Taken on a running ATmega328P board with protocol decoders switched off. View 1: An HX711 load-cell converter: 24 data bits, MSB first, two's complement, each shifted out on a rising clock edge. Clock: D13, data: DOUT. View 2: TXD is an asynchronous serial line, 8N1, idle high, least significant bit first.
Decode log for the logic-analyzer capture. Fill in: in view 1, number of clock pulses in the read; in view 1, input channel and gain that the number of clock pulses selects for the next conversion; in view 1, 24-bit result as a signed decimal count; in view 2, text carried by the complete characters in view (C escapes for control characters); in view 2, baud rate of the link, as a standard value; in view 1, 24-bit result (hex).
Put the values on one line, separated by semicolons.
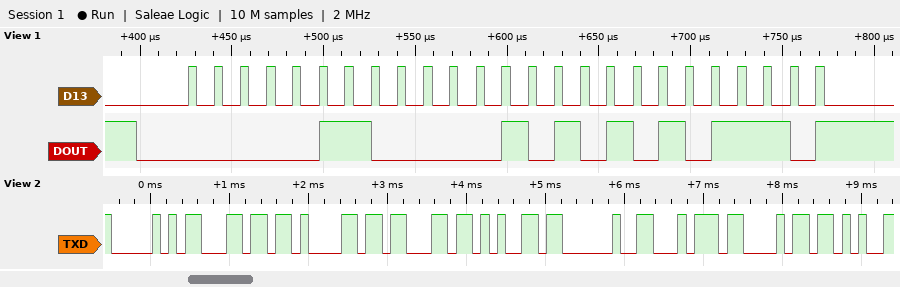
25; channel A, gain 128; 395950; "Place th"; 9600 baud; 0x060AAE
